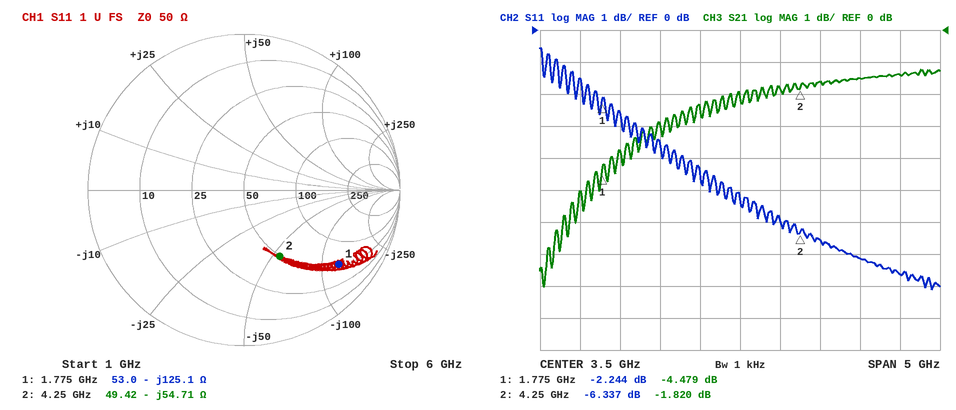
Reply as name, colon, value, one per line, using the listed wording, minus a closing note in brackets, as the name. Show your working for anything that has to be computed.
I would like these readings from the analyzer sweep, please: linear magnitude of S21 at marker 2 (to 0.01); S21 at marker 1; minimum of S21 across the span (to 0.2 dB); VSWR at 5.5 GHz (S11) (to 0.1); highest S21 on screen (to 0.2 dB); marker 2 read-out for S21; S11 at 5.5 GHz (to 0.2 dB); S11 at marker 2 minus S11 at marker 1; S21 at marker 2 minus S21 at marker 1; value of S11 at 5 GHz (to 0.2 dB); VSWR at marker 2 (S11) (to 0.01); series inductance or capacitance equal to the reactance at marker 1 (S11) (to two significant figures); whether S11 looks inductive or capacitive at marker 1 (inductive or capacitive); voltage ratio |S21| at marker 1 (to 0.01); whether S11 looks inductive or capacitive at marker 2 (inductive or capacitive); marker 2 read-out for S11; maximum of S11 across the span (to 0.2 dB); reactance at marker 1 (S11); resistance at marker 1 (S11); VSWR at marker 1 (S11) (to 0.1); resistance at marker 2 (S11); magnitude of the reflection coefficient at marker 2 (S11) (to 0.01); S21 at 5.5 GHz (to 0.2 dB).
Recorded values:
linear magnitude of S21 at marker 2: 10^(-1.82/20) ≈ 0.81
S21 at marker 1: -4.479 dB
minimum of S21 across the span: -8.0 dB
VSWR at 5.5 GHz (S11): |Γ| = 10^(-7.6/20) = 0.4169; VSWR = (1 + 0.4169)/(1 − 0.4169) ≈ 2.4
highest S21 on screen: -1.2 dB
marker 2 read-out for S21: -1.820 dB
S11 at 5.5 GHz: -7.6 dB
S11 at marker 2 minus S11 at marker 1: -6.337 − (-2.244) = -4.093 dB
S21 at marker 2 minus S21 at marker 1: -1.82 − (-4.479) = 2.659 dB
value of S11 at 5 GHz: -7.2 dB
VSWR at marker 2 (S11): (1 + 0.4821)/(1 − 0.4821) ≈ 2.86
series inductance or capacitance equal to the reactance at marker 1 (S11): C = 1/(2π × 1.775 GHz × 125.1 Ω) ≈ 717 fF, so 720 fF to two significant figures
whether S11 looks inductive or capacitive at marker 1: capacitive
voltage ratio |S21| at marker 1: 10^(-4.479/20) ≈ 0.60
whether S11 looks inductive or capacitive at marker 2: capacitive
marker 2 read-out for S11: -6.337 dB
maximum of S11 across the span: -0.6 dB
reactance at marker 1: -125.1 Ω
resistance at marker 1: 53.0 Ω
VSWR at marker 1 (S11): 7.8
resistance at marker 2: 49.42 Ω
magnitude of the reflection coefficient at marker 2 (S11): 0.48
S21 at 5.5 GHz: -1.4 dB
